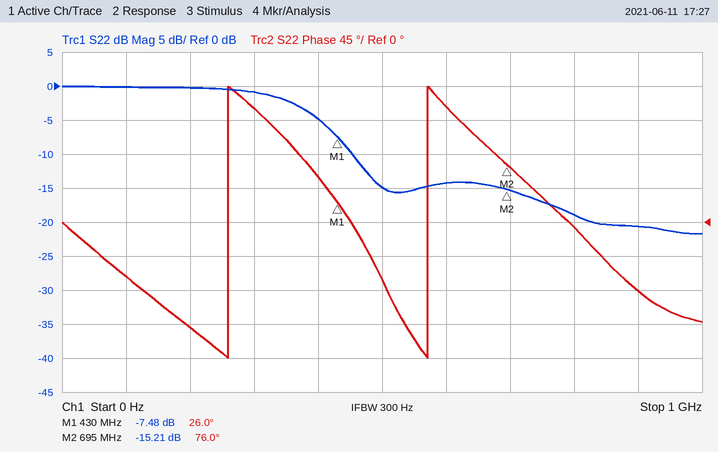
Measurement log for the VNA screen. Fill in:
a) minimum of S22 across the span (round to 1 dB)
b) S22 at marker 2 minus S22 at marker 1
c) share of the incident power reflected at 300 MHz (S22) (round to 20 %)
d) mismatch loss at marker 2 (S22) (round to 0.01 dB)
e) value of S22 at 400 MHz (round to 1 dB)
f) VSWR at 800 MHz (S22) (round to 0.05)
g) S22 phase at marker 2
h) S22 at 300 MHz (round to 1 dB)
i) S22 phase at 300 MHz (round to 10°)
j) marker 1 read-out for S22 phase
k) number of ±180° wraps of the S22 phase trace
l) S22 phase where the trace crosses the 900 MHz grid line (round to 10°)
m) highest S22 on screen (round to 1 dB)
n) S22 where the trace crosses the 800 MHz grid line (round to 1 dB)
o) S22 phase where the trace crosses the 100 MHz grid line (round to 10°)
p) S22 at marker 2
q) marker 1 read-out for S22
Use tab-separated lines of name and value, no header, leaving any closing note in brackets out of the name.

minimum of S22 across the span	-22 dB
S22 at marker 2 minus S22 at marker 1	-7.73 dB
share of the incident power reflected at 300 MHz (S22)	80 %
mismatch loss at marker 2 (S22)	0.13 dB
value of S22 at 400 MHz	-5 dB
VSWR at 800 MHz (S22)	1.25
S22 phase at marker 2	76.0°
S22 at 300 MHz	-1 dB
S22 phase at 300 MHz	150°
marker 1 read-out for S22 phase	26.0°
number of ±180° wraps of the S22 phase trace	2
S22 phase where the trace crosses the 900 MHz grid line	-90°
highest S22 on screen	0 dB
S22 where the trace crosses the 800 MHz grid line	-19 dB
S22 phase where the trace crosses the 100 MHz grid line	-70°
S22 at marker 2	-15.21 dB
marker 1 read-out for S22	-7.48 dB
